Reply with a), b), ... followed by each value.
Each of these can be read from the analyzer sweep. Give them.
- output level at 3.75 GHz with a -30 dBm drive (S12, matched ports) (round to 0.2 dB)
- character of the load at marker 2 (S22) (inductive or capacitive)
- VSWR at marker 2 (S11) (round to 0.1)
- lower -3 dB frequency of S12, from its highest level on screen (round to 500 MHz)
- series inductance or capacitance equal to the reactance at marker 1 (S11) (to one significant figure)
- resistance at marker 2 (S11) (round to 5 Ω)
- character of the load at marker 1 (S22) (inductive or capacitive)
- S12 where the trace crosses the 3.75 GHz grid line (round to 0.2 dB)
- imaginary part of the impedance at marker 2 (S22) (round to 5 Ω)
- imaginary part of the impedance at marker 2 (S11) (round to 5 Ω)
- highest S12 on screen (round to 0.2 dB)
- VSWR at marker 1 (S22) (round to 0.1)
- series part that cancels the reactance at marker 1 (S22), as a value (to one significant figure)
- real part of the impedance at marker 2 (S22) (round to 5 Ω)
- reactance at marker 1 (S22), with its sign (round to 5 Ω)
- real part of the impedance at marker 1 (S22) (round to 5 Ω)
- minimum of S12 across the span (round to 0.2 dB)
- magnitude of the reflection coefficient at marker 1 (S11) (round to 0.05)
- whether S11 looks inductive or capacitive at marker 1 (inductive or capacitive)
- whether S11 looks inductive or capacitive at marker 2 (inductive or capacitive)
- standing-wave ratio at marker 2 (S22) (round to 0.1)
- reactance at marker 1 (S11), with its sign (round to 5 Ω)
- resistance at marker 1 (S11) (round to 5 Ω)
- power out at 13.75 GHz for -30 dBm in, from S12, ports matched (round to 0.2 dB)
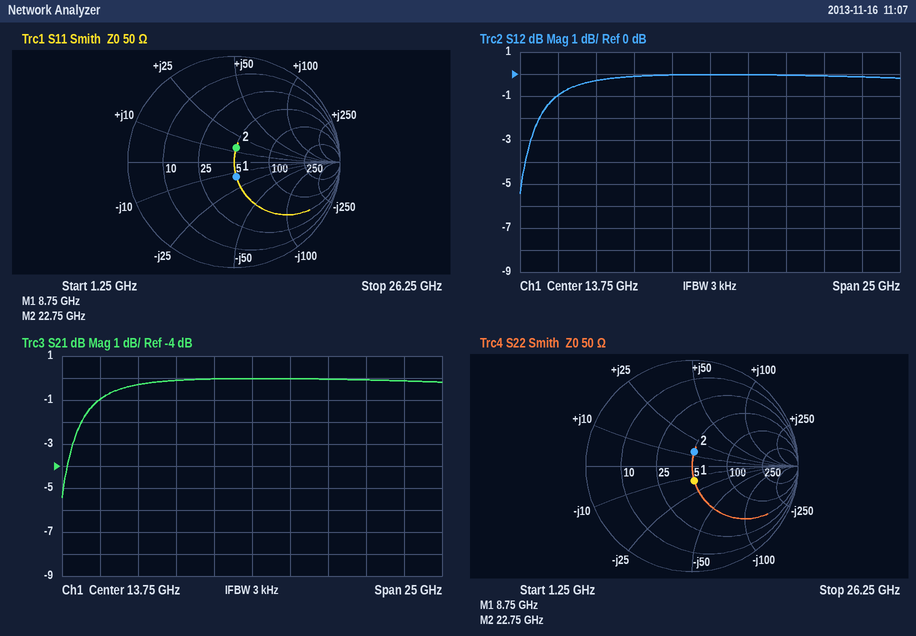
a) -31.0 dBm
b) inductive
c) 1.3
d) 2.0 GHz
e) 1 pF
f) 50 Ω
g) capacitive
h) -1.0 dB
i) +15 Ω
j) +15 Ω
k) 0.0 dB
l) 1.3
m) 300 pH
n) 50 Ω
o) -15 Ω
p) 50 Ω
q) -5.4 dB
r) 0.15
s) capacitive
t) inductive
u) 1.3
v) -15 Ω
w) 50 Ω
x) -30.0 dBm
